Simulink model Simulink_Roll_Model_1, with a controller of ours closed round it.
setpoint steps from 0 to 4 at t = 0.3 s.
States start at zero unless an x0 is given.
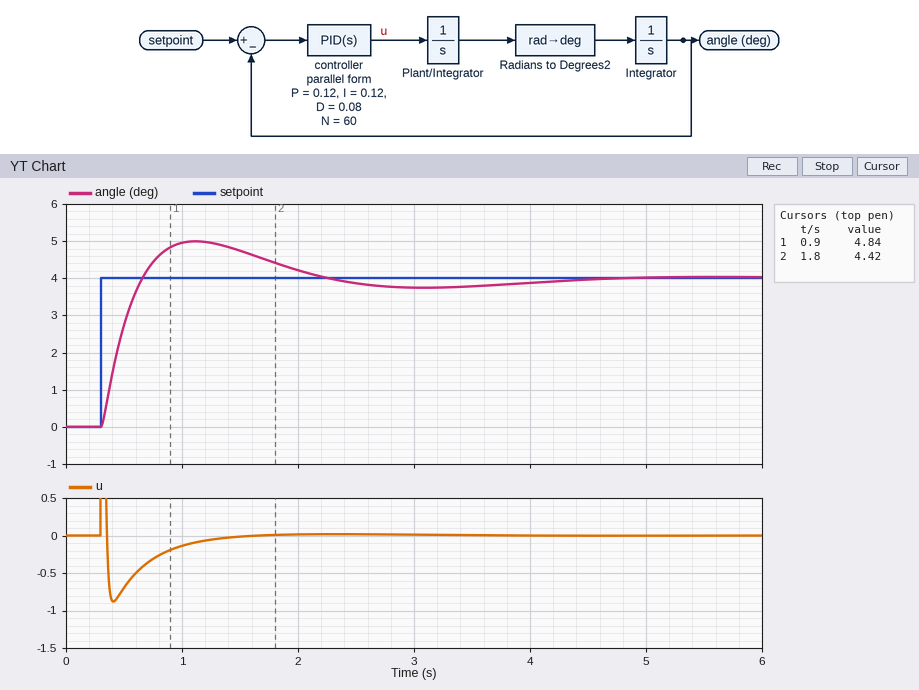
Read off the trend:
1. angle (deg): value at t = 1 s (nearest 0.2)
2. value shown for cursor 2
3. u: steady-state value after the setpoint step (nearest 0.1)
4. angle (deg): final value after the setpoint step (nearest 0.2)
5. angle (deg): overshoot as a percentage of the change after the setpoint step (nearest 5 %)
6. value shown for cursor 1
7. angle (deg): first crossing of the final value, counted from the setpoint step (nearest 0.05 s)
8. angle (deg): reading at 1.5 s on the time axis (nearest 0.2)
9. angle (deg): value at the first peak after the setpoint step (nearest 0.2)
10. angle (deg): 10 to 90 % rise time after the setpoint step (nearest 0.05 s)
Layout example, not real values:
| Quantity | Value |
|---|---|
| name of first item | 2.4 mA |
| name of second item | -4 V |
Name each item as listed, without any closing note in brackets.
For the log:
| Quantity | Value |
|---|---|
| angle (deg): value at t = 1 s | 5.0 |
| value shown for cursor 2 | 4.42 |
| u: steady-state value after the setpoint step | 0.0 |
| angle (deg): final value after the setpoint step | 4.0 |
| angle (deg): overshoot as a percentage of the change after the setpoint step | 25 % |
| value shown for cursor 1 | 4.84 |
| angle (deg): first crossing of the final value, counted from the setpoint step | 0.35 s |
| angle (deg): reading at 1.5 s on the time axis | 4.8 |
| angle (deg): value at the first peak after the setpoint step | 5.0 |
| angle (deg): 10 to 90 % rise time after the setpoint step | 0.25 s |
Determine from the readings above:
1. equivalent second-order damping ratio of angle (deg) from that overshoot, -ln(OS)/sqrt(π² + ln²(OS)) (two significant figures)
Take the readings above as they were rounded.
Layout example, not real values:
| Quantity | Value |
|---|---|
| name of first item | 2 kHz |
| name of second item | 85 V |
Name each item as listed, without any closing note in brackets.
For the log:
| Quantity | Value |
|---|---|
| equivalent second-order damping ratio of angle (deg) from that overshoot, -ln(OS)/sqrt(π² + ln²(OS)) | 0.40 |
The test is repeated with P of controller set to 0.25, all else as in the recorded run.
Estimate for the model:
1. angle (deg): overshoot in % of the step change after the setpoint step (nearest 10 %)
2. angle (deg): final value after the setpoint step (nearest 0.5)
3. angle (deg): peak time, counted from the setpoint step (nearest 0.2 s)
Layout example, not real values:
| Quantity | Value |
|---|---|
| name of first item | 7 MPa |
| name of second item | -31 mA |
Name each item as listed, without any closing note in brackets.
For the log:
| Quantity | Value |
|---|---|
| angle (deg): overshoot in % of the step change after the setpoint step | 30 % |
| angle (deg): final value after the setpoint step | 4.0 |
| angle (deg): peak time, counted from the setpoint step | 0.6 s |
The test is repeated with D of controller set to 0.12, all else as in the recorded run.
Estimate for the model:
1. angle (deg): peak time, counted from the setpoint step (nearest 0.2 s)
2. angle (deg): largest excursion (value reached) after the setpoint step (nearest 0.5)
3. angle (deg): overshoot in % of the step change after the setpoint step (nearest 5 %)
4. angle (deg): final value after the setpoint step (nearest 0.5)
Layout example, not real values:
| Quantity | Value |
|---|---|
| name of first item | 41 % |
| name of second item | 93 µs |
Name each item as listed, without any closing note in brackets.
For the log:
| Quantity | Value |
|---|---|
| angle (deg): peak time, counted from the setpoint step | 0.8 s |
| angle (deg): largest excursion (value reached) after the setpoint step | 4.5 |
| angle (deg): overshoot in % of the step change after the setpoint step | 15 % |
| angle (deg): final value after the setpoint step | 4.0 |
